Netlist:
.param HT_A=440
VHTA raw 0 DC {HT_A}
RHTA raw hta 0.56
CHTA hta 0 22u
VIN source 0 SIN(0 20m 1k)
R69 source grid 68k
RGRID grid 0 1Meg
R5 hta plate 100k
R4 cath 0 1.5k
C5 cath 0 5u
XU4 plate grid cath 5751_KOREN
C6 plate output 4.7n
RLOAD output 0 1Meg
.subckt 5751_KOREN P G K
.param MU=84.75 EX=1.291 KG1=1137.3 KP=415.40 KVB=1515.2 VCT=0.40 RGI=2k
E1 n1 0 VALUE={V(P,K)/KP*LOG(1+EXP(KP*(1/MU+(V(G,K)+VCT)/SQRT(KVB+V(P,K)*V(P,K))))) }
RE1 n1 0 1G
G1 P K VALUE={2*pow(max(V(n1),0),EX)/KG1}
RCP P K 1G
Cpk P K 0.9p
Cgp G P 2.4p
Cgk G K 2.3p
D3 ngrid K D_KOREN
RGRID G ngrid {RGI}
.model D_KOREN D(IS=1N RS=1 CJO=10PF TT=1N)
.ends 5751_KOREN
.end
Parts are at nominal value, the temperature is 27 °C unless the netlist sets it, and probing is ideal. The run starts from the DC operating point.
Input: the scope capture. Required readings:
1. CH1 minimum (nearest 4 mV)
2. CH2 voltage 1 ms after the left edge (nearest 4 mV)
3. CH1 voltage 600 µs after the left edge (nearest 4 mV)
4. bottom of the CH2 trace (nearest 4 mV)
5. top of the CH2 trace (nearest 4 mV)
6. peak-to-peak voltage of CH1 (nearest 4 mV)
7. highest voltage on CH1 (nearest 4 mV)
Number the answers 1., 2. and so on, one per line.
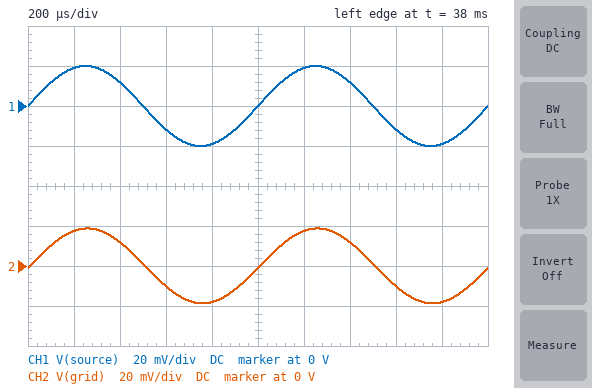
1. -20 mV
2. 0 V
3. -12 mV
4. -20 mV
5. 20 mV
6. 40 mV
7. 20 mV
